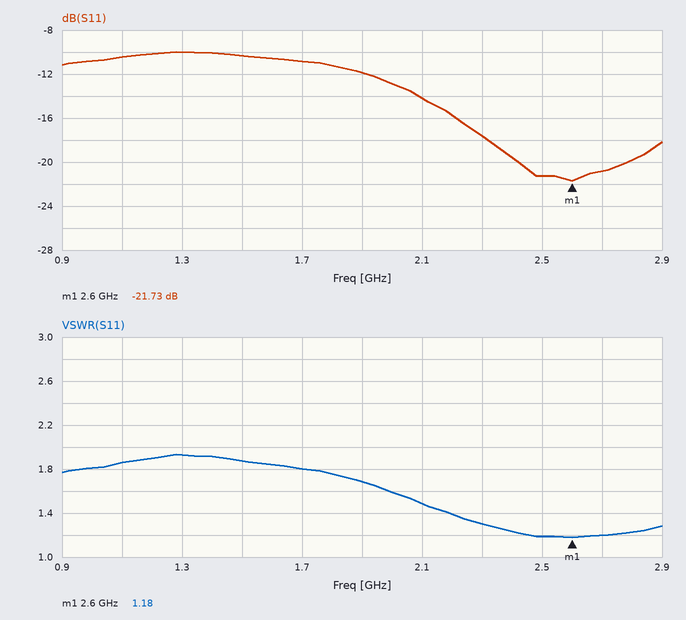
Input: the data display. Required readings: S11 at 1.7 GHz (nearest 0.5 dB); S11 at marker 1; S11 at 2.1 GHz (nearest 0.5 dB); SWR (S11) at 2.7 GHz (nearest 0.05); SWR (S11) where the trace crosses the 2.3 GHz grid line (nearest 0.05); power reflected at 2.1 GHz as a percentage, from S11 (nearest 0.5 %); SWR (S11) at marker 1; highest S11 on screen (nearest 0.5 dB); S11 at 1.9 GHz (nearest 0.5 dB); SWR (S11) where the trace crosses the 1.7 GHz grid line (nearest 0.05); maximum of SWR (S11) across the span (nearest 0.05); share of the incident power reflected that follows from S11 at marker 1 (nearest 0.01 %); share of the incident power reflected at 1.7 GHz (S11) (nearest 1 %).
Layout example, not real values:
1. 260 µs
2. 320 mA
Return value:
1. -11.0 dB
2. -21.73 dB
3. -14.0 dB
4. 1.20
5. 1.30
6. 4.0 %
7. 1.18
8. -10.0 dB
9. -12.0 dB
10. 1.80
11. 1.95
12. 0.67 %
13. 8 %
